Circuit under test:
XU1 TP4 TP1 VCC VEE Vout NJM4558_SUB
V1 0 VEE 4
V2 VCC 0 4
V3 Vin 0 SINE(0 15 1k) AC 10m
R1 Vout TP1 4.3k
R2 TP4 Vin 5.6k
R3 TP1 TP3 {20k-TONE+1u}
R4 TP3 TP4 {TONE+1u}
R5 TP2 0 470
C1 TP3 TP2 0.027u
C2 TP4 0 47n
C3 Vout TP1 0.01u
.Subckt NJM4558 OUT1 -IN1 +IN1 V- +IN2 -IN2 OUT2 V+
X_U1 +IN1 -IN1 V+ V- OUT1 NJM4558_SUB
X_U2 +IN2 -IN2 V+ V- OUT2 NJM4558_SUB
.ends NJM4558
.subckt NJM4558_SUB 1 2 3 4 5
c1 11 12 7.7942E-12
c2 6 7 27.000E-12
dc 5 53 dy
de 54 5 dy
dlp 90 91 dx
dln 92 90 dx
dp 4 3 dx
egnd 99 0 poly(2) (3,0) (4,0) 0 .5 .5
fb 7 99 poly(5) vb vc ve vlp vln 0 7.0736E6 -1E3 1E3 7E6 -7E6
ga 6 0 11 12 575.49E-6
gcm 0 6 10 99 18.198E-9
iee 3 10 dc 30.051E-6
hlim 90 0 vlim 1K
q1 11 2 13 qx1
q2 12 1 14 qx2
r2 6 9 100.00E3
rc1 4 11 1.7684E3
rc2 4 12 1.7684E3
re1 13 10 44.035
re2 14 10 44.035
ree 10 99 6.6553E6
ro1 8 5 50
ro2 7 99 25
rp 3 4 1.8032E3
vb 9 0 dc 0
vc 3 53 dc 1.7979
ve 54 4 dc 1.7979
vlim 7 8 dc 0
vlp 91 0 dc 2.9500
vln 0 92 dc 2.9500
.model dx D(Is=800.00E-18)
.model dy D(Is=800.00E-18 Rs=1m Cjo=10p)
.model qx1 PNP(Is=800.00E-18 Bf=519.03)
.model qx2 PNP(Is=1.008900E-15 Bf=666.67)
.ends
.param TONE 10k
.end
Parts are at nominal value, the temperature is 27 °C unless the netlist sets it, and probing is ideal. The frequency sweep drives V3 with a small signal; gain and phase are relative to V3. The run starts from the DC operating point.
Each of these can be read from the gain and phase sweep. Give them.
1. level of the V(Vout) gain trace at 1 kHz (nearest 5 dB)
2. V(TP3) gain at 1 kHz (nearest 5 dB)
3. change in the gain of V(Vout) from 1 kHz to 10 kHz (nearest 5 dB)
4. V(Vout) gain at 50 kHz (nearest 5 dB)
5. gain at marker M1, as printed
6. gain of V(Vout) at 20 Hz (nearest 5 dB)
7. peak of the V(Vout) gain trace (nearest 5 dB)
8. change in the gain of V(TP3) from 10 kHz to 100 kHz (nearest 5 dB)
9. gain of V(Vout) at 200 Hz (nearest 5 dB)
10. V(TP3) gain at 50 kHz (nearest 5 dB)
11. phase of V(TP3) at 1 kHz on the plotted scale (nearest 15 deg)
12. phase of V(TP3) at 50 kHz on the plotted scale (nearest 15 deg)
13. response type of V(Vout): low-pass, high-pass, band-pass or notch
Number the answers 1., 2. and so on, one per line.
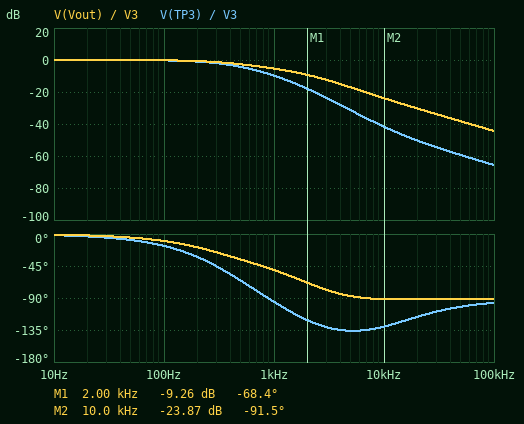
1. -5 dB
2. -10 dB
3. -20 dB
4. -40 dB
5. -9.26 dB
6. 0 dB
7. 0 dB
8. -25 dB
9. 0 dB
10. -60 dB
11. -90 deg
12. -105 deg
13. low-pass
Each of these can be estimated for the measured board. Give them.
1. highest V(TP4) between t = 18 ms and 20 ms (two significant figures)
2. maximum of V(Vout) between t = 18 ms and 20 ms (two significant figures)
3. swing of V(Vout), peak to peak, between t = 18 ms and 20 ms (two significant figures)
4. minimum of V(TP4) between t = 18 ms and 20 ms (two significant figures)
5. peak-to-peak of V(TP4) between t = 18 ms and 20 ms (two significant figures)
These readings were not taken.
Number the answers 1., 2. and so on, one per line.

1. 7.0 V
2. 3.0 V
3. 5.9 V
4. -5.6 V
5. 13 V
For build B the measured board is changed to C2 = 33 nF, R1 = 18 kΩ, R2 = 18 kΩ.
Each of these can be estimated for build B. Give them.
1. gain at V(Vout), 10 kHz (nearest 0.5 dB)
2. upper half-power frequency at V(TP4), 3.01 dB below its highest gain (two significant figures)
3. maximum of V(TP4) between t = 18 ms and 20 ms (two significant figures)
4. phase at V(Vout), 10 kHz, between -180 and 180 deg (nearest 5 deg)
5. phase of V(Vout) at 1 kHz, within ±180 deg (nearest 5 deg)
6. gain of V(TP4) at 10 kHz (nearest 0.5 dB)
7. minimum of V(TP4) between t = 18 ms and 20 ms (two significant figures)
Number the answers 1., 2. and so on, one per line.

1. -31.0 dB
2. 180 Hz
3. 3.1 V
4. -95 deg
5. -70 deg
6. -31.5 dB
7. -3.1 V
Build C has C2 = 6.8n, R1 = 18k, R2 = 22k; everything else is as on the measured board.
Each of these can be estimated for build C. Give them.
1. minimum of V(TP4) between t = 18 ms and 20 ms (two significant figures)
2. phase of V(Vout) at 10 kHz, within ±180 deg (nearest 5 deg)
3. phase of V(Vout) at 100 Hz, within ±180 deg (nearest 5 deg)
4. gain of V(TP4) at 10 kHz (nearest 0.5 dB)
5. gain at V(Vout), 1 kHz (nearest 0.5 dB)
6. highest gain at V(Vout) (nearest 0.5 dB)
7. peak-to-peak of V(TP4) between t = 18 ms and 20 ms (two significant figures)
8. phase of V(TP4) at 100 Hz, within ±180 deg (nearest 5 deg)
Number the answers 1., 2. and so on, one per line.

1. -4.7 V
2. -80 deg
3. -5 deg
4. -20.0 dB
5. -4.0 dB
6. 0 dB
7. 9.9 V
8. -15 deg
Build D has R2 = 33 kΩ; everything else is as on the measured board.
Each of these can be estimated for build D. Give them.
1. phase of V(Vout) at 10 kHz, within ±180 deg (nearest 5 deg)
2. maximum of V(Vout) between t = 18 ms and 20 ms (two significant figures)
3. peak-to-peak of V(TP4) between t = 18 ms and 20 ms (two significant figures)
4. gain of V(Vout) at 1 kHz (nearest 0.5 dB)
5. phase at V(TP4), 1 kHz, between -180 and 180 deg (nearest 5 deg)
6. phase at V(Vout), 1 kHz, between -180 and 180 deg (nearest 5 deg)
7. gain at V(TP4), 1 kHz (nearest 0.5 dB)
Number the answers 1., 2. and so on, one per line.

1. -95 deg
2. 1.6 V
3. 2.6 V
4. -19.5 dB
5. -80 deg
6. -70 deg
7. -21.0 dB
